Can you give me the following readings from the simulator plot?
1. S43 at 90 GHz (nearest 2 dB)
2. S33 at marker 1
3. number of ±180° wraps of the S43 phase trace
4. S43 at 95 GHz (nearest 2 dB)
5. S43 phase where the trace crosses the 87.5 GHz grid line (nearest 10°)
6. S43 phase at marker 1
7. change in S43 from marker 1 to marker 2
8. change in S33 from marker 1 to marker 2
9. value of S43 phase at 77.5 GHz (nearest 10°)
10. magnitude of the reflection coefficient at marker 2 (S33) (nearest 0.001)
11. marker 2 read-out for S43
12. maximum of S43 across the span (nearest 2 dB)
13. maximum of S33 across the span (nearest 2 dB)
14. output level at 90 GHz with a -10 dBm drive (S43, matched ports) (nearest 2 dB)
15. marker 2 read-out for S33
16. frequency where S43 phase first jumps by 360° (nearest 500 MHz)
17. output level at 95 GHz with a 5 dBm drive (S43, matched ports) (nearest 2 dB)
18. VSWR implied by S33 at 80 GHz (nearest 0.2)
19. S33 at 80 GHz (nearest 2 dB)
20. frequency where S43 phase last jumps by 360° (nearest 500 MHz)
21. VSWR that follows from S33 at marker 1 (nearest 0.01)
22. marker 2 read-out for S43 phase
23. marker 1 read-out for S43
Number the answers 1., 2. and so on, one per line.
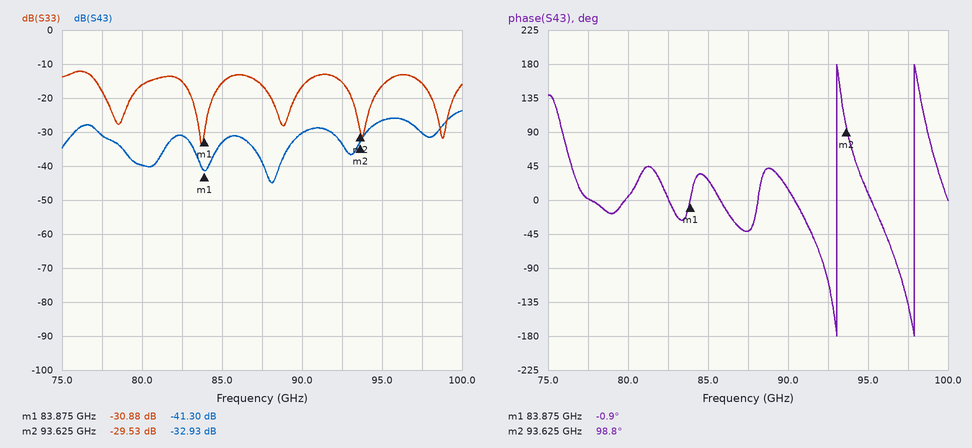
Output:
1. -30 dB
2. -30.88 dB
3. 2
4. -26 dB
5. -40°
6. -0.9°
7. 8.37 dB
8. 1.35 dB
9. 0°
10. 0.033
11. -32.93 dB
12. -24 dB
13. -12 dB
14. -40 dBm
15. -29.53 dB
16. 93.0 GHz
17. -22 dBm
18. 1.4
19. -16 dB
20. 98.0 GHz
21. 1.06
22. 98.8°
23. -41.30 dB
